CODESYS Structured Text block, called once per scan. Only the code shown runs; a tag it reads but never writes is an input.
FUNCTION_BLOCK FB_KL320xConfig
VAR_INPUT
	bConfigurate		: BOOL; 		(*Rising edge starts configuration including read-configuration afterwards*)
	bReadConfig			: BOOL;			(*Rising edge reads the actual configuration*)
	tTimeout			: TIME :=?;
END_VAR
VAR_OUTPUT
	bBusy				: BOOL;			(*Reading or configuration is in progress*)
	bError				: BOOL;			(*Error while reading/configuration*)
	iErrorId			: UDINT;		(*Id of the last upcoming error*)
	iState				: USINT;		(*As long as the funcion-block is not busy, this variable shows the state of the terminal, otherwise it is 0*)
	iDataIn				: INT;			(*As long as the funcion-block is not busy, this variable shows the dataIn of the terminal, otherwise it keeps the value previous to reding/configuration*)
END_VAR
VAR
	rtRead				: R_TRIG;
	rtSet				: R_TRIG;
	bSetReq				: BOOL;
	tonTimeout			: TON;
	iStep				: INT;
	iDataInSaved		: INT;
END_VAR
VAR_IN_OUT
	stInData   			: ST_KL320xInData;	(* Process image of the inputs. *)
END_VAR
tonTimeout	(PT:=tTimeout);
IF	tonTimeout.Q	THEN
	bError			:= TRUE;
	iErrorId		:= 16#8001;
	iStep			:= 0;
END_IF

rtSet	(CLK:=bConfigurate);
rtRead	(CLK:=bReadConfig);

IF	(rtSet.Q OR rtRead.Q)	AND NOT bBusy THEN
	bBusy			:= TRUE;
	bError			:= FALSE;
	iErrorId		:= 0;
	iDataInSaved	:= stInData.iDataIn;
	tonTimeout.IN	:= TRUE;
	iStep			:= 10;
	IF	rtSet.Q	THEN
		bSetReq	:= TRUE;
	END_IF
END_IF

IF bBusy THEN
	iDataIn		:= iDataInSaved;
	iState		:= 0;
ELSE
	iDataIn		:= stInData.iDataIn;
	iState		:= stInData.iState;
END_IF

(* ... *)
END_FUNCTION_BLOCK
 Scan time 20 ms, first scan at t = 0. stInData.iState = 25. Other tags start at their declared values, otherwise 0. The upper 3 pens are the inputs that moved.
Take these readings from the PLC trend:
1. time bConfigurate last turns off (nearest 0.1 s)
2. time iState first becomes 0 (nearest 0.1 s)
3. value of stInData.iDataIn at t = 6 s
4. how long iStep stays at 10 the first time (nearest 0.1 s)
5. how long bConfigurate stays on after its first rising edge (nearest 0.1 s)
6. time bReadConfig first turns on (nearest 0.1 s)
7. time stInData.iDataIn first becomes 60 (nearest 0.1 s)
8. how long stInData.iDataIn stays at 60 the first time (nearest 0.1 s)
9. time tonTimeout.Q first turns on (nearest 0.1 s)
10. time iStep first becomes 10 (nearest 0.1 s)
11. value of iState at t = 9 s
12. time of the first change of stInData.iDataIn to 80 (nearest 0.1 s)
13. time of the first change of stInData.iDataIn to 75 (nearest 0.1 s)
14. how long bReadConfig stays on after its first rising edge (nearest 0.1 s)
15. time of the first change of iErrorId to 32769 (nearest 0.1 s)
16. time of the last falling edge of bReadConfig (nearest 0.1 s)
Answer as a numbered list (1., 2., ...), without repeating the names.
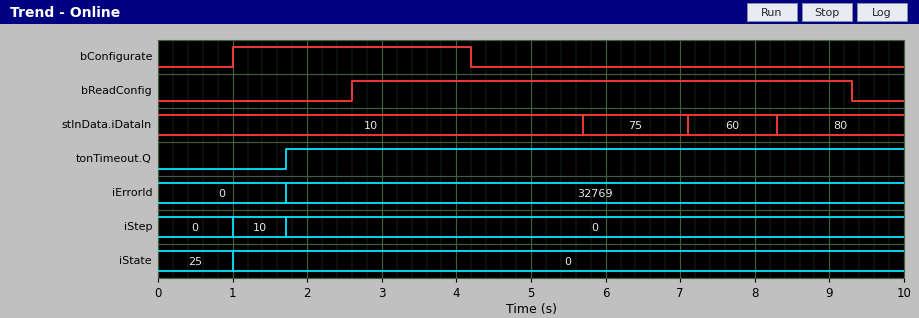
1. 4.2 s
2. 1.0 s
3. 75
4. 0.7 s
5. 3.2 s
6. 2.6 s
7. 7.1 s
8. 1.2 s
9. 1.7 s
10. 1.0 s
11. 0
12. 8.3 s
13. 5.7 s
14. 6.7 s
15. 1.7 s
16. 9.3 s
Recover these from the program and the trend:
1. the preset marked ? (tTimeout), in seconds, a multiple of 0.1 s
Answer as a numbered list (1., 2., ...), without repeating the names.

1. 0.7 s
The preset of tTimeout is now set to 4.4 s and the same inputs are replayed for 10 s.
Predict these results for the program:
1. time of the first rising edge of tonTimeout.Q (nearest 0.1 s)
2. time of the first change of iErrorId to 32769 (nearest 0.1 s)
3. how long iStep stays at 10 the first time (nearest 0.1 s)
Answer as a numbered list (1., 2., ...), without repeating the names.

1. 5.4 s
2. 5.4 s
3. 4.4 s
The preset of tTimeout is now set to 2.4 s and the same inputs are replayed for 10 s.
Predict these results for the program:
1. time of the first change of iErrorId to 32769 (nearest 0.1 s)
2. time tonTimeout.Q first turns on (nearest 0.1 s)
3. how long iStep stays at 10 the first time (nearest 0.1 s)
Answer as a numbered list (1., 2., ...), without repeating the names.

1. 3.4 s
2. 3.4 s
3. 2.4 s
